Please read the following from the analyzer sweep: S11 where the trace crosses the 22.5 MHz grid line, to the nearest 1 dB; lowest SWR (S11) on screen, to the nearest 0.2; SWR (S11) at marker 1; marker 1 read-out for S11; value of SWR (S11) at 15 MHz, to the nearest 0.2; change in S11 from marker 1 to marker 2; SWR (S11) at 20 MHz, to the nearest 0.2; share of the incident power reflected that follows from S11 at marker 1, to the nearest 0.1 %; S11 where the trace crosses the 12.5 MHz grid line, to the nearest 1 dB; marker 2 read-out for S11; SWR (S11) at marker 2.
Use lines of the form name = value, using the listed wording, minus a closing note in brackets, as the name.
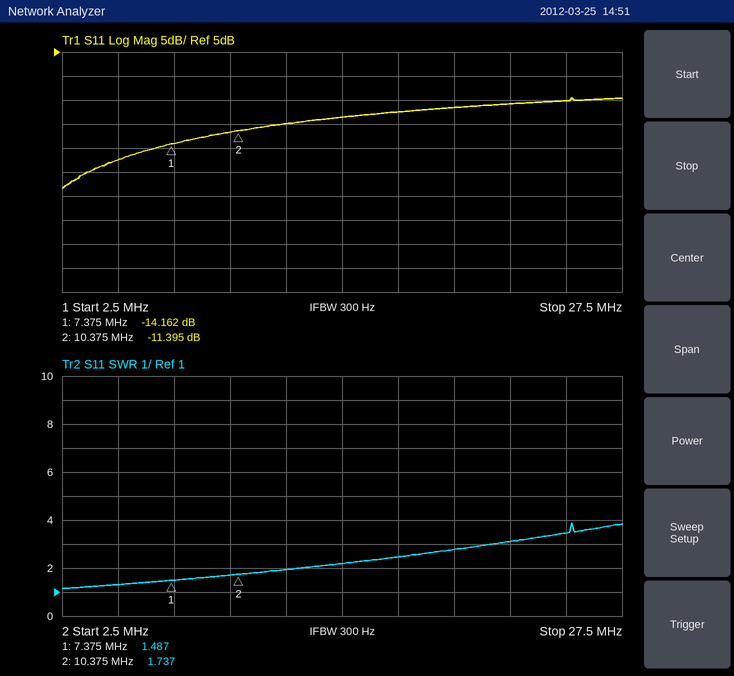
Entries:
S11 where the trace crosses the 22.5 MHz grid line, to the nearest 1 dB = -6 dB
lowest SWR (S11) on screen, to the nearest 0.2 = 1.2
SWR (S11) at marker 1 = 1.487
marker 1 read-out for S11 = -14.162 dB
value of SWR (S11) at 15 MHz, to the nearest 0.2 = 2.2
change in S11 from marker 1 to marker 2 = 2.767 dB
SWR (S11) at 20 MHz, to the nearest 0.2 = 2.8
share of the incident power reflected that follows from S11 at marker 1, to the nearest 0.1 % = 3.8 %
S11 where the trace crosses the 12.5 MHz grid line, to the nearest 1 dB = -10 dB
marker 2 read-out for S11 = -11.395 dB
SWR (S11) at marker 2 = 1.737
